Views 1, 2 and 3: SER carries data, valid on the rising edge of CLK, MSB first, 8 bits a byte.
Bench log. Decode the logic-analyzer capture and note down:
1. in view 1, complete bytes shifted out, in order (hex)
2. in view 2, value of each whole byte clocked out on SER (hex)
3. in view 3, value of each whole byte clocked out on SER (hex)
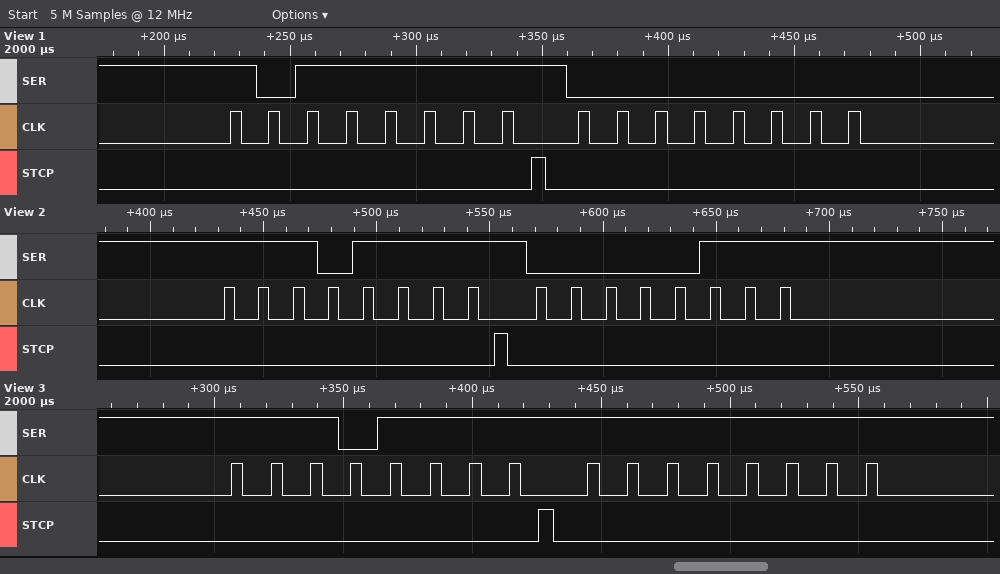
0xBF 0x00
0xEF 0x07
EF FF
